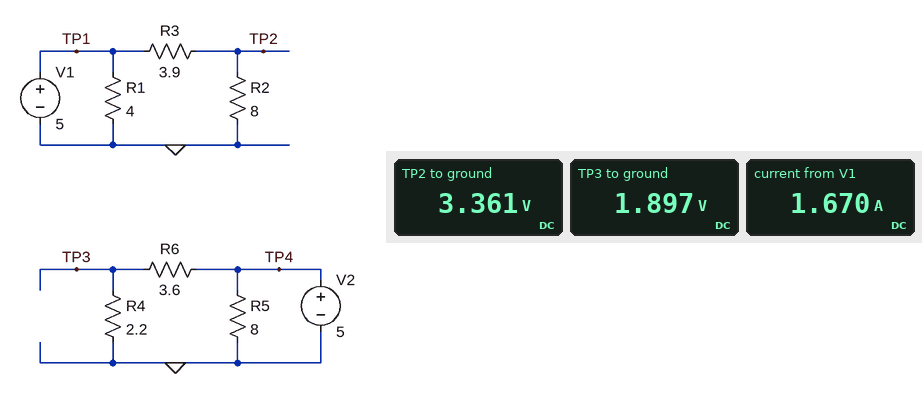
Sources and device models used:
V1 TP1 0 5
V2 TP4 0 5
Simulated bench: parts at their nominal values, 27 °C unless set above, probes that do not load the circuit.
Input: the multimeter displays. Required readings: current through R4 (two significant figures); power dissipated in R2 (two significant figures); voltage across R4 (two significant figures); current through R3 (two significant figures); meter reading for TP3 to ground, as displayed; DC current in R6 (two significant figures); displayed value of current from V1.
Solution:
860 mA
1.4 W
1.9 V
420 mA
1.897 V
860 mA
1.670 A
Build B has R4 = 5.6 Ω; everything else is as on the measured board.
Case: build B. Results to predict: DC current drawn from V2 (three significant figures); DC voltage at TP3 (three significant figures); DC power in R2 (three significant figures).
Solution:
1.17 A
3.04 V
1.41 W
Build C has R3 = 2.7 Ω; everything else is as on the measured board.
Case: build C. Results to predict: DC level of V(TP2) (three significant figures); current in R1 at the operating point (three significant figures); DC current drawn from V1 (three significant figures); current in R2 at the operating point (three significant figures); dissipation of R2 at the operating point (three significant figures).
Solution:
3.74 V
1.25 A
1.72 A
467 mA
1.75 W
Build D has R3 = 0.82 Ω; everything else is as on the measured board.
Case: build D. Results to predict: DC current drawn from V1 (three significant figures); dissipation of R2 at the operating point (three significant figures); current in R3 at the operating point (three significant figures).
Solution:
1.82 A
2.57 W
567 mA
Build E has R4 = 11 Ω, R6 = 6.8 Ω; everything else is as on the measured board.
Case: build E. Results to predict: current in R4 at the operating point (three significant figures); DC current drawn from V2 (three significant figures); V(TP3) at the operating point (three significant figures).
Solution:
281 mA
906 mA
3.09 V
